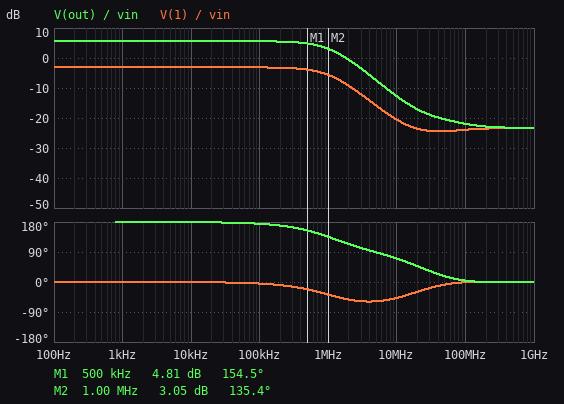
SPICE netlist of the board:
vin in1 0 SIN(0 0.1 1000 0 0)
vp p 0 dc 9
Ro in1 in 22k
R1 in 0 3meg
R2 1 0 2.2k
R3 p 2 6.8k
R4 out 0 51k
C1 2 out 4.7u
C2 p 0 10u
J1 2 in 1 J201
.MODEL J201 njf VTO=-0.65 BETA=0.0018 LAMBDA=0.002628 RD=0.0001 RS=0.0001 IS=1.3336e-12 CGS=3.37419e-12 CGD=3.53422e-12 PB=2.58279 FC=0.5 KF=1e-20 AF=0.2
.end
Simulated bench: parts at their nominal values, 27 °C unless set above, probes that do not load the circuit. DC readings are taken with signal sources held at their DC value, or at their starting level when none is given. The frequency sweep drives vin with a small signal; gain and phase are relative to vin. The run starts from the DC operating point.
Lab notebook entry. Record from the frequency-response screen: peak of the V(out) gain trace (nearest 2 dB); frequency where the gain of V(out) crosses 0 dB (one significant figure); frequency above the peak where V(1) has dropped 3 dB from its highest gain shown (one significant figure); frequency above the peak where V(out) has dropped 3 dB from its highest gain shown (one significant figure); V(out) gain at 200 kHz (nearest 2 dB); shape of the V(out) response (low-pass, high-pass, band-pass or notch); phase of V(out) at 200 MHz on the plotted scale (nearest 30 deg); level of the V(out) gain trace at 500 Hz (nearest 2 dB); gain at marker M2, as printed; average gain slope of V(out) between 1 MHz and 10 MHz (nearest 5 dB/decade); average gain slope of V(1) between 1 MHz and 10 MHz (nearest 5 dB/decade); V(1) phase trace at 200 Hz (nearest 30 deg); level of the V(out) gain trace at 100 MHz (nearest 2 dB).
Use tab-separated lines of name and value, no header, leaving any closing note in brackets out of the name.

peak of the V(out) gain trace	6 dB
frequency where the gain of V(out) crosses 0 dB	2 MHz
frequency above the peak where V(1) has dropped 3 dB from its highest gain shown	1 MHz
frequency above the peak where V(out) has dropped 3 dB from its highest gain shown	1 MHz
V(out) gain at 200 kHz	6 dB
shape of the V(out) response	low-pass
phase of V(out) at 200 MHz on the plotted scale	0 deg
level of the V(out) gain trace at 500 Hz	6 dB
gain at marker M2, as printed	3.05 dB
average gain slope of V(out) between 1 MHz and 10 MHz	-15 dB/decade
average gain slope of V(1) between 1 MHz and 10 MHz	-15 dB/decade
V(1) phase trace at 200 Hz	0 deg
level of the V(out) gain trace at 100 MHz	-22 dB
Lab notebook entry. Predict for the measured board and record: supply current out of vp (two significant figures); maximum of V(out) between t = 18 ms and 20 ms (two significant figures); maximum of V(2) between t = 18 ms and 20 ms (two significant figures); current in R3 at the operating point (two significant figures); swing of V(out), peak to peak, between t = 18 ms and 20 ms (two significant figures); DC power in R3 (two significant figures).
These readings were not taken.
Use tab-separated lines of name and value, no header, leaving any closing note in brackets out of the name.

supply current out of vp	160 µA
maximum of V(out) between t = 18 ms and 20 ms	190 mV
maximum of V(2) between t = 18 ms and 20 ms	8.1 V
current in R3 at the operating point	160 µA
swing of V(out), peak to peak, between t = 18 ms and 20 ms	380 mV
DC power in R3	180 µW
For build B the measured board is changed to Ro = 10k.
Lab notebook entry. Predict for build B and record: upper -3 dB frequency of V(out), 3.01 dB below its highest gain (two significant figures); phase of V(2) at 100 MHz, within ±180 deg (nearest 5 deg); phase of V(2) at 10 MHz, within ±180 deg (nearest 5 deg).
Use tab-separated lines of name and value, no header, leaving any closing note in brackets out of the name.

upper -3 dB frequency of V(out), 3.01 dB below its highest gain	2.3 MHz
phase of V(2) at 100 MHz, within ±180 deg	5 deg
phase of V(2) at 10 MHz, within ±180 deg	75 deg
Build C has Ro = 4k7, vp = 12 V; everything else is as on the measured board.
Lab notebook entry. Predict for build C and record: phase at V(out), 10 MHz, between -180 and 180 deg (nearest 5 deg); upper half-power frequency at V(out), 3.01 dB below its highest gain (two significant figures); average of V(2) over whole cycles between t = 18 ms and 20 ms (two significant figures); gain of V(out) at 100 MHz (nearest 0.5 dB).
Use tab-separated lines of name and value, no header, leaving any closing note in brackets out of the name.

phase at V(out), 10 MHz, between -180 and 180 deg	90 deg
upper half-power frequency at V(out), 3.01 dB below its highest gain	4.7 MHz
average of V(2) over whole cycles between t = 18 ms and 20 ms	11 V
gain of V(out) at 100 MHz	-10.5 dB
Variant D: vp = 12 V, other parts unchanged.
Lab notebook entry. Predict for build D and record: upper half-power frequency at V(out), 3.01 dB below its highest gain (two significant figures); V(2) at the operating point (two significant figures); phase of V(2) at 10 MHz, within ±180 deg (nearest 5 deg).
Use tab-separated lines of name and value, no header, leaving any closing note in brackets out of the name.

upper half-power frequency at V(out), 3.01 dB below its highest gain	1.2 MHz
V(2) at the operating point	11 V
phase of V(2) at 10 MHz, within ±180 deg	75 deg
